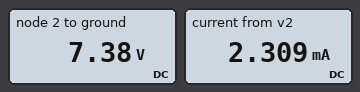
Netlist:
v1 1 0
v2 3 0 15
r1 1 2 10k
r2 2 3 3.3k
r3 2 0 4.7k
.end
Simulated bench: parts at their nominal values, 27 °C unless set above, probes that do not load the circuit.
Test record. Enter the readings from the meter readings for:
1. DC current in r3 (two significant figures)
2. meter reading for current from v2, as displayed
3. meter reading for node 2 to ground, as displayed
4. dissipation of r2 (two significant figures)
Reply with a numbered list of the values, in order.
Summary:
1. 1.6 mA
2. 2.309 mA
3. 7.38 V
4. 18 mW
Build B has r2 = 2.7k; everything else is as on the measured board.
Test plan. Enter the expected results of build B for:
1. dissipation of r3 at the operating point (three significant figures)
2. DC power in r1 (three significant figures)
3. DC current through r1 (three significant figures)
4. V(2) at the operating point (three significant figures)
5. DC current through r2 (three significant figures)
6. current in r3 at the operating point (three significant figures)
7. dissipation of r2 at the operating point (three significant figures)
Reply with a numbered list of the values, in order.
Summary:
1. 14.1 mW
2. 6.61 mW
3. 813 µA
4. 8.13 V
5. 2.54 mA
6. 1.73 mA
7. 17.5 mW
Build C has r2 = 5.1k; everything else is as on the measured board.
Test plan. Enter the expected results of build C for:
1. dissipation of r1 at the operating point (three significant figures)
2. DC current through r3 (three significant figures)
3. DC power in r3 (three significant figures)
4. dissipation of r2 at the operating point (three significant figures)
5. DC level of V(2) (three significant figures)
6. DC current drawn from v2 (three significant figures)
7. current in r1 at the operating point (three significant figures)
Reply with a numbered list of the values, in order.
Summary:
1. 3.34 mW
2. 1.23 mA
3. 7.11 mW
4. 16.7 mW
5. 5.78 V
6. 1.81 mA
7. 578 µA
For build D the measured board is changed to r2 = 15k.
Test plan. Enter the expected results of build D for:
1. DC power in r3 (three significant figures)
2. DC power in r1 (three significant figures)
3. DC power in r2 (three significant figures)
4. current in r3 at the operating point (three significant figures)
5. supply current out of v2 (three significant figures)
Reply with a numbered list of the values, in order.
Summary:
1. 1.48 mW
2. 695 µW
3. 10.2 mW
4. 561 µA
5. 824 µA
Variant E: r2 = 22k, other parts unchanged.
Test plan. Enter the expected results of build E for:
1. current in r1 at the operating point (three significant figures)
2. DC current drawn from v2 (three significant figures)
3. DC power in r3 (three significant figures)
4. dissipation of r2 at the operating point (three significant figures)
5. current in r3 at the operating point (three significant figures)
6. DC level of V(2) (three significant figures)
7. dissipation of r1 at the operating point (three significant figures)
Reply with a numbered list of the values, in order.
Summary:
1. 190 µA
2. 595 µA
3. 771 µW
4. 7.80 mW
5. 405 µA
6. 1.90 V
7. 362 µW
